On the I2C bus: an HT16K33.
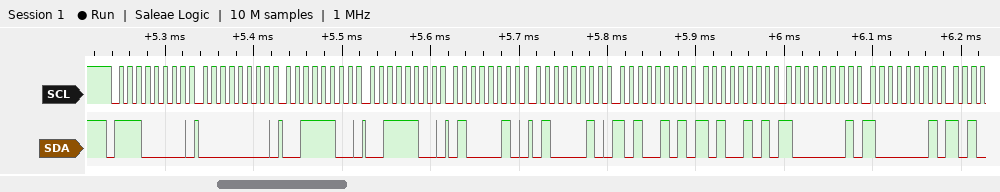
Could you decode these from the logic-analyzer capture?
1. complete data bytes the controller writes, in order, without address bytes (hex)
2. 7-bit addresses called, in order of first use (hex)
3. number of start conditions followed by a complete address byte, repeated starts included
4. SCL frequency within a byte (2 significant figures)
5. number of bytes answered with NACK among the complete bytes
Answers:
00 3C 3C 42 42 A5 A5 81 81
0x70
1
100 kHz
0
